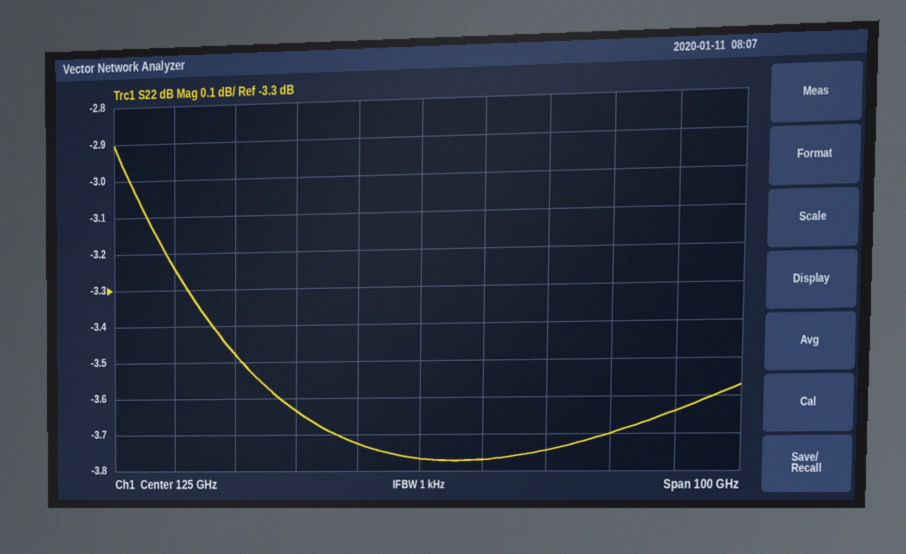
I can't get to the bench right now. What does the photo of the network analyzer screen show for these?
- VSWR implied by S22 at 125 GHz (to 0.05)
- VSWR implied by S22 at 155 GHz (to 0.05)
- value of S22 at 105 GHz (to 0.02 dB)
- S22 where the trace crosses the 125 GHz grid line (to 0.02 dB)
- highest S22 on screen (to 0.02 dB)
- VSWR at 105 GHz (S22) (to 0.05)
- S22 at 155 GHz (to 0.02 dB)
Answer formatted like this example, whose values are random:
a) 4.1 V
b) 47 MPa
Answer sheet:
a) 4.70
b) 4.75
c) -3.64 dB
d) -3.76 dB
e) -2.90 dB
f) 4.85
g) -3.70 dB
